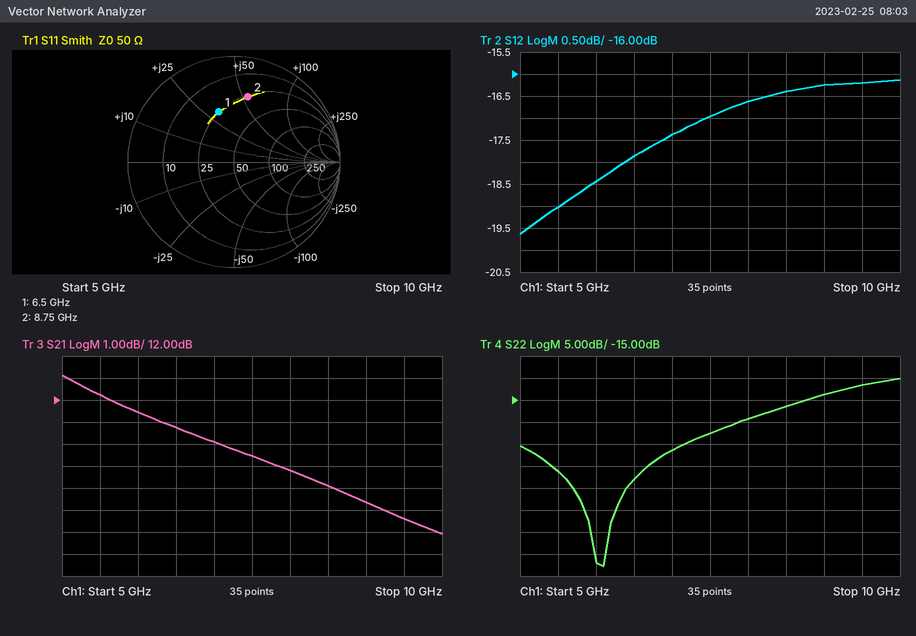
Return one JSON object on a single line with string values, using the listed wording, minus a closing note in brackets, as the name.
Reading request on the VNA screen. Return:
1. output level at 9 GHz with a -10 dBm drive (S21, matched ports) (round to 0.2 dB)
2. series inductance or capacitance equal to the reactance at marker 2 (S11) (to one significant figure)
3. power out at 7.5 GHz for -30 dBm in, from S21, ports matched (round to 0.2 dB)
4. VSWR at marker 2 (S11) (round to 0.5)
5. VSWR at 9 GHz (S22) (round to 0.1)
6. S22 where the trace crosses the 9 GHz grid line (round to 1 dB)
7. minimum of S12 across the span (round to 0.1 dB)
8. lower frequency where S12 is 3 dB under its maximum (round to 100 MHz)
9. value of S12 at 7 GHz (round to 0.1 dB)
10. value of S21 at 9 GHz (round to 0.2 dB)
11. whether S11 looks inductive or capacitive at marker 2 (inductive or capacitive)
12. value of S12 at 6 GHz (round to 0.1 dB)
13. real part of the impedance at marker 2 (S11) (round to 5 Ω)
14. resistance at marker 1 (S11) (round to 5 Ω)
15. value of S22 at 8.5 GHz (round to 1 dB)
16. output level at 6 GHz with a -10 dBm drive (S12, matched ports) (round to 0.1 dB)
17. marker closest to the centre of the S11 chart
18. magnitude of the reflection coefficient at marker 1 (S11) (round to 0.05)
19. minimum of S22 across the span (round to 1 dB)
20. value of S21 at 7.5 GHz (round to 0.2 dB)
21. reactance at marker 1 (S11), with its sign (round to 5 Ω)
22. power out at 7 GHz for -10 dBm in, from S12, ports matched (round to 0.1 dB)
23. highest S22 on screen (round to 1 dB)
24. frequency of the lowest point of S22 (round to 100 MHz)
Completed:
{"output level at 9 GHz with a -10 dBm drive (S21, matched ports)": "-2.6 dBm", "series inductance or capacitance equal to the reactance at marker 2 (S11)": "1.0 nH", "power out at 7.5 GHz for -30 dBm in, from S21, ports matched": "-20.6 dBm", "VSWR at marker 2 (S11)": "4.5", "VSWR at 9 GHz (S22)": "1.5", "S22 where the trace crosses the 9 GHz grid line": "-14 dB", "minimum of S12 across the span": "-19.6 dB", "lower frequency where S12 is 3 dB under its maximum": "5.4 GHz", "value of S12 at 7 GHz": "-17.4 dB", "value of S21 at 9 GHz": "7.4 dB", "whether S11 looks inductive or capacitive at marker 2": "inductive", "value of S12 at 6 GHz": "-18.4 dB", "real part of the impedance at marker 2 (S11)": "25 Ω", "resistance at marker 1 (S11)": "25 Ω", "value of S22 at 8.5 GHz": "-16 dB", "output level at 6 GHz with a -10 dBm drive (S12, matched ports)": "-28.4 dBm", "marker closest to the centre of the S11 chart": "marker 1", "magnitude of the reflection coefficient at marker 1 (S11)": "0.50", "minimum of S22 across the span": "-53 dB", "value of S21 at 7.5 GHz": "9.4 dB", "reactance at marker 1 (S11), with its sign": "+30 Ω", "power out at 7 GHz for -10 dBm in, from S12, ports matched": "-27.4 dBm", "highest S22 on screen": "-10 dB", "frequency of the lowest point of S22": "6.1 GHz"}
